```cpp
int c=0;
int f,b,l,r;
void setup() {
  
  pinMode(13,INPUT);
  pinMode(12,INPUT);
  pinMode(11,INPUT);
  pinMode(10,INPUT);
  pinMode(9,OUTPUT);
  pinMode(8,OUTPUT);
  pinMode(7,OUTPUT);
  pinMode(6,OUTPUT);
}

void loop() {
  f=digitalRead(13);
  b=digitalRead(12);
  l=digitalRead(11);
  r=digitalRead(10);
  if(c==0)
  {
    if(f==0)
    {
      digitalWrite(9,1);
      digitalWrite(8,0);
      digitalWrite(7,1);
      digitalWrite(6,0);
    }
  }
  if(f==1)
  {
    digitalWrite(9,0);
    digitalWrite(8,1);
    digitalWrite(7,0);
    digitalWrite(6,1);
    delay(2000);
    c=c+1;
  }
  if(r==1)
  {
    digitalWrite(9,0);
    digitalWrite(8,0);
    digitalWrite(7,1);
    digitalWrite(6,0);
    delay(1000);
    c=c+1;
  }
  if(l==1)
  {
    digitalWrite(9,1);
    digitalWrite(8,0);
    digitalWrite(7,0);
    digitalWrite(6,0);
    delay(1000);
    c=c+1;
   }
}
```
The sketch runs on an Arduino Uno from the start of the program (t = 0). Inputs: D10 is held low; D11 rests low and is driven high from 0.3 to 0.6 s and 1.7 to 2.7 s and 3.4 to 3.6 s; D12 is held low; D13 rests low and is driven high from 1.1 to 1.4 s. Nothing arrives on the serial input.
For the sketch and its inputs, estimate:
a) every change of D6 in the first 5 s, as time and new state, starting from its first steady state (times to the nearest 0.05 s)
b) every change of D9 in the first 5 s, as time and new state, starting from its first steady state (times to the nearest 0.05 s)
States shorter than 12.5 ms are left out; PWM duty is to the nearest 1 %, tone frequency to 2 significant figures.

0 s low; 1.3 s high; 3.4 s low
0 s high; 1.3 s low; 3.4 s high
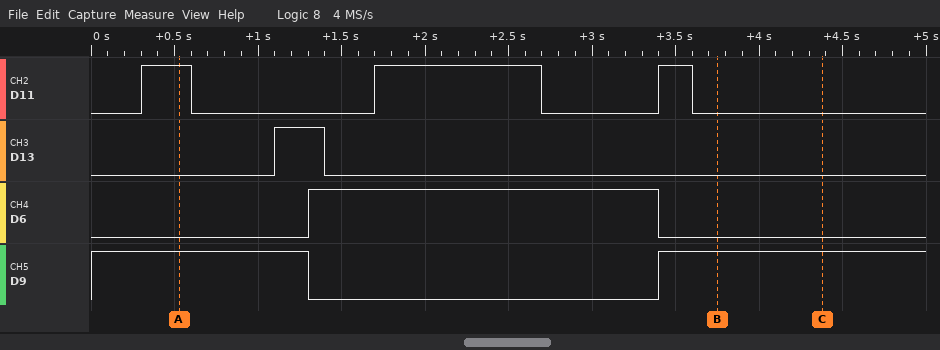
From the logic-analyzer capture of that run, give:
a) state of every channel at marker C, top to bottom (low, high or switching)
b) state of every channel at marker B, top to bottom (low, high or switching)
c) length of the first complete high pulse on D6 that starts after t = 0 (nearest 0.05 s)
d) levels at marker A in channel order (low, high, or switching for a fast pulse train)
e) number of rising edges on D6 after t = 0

D11 low, D13 low, D6 low, D9 high
D11 low, D13 low, D6 low, D9 high
2.10 s
D11 high, D13 low, D6 low, D9 high
1
